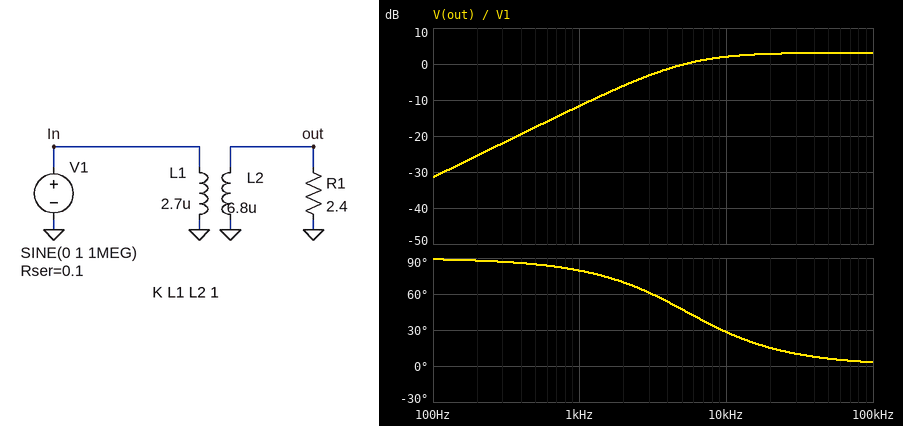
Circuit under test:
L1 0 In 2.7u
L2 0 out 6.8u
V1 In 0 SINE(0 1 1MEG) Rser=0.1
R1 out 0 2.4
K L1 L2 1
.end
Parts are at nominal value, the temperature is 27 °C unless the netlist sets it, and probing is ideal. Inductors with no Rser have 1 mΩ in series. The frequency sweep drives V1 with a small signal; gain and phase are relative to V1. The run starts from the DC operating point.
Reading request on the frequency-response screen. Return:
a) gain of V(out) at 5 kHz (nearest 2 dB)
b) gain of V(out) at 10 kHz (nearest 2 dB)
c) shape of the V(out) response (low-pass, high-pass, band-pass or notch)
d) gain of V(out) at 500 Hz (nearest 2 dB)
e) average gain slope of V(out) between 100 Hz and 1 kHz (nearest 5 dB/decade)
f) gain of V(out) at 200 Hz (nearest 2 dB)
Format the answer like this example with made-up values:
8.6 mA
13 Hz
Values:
0 dB
2 dB
high-pass
-18 dB
20 dB/decade
-26 dB
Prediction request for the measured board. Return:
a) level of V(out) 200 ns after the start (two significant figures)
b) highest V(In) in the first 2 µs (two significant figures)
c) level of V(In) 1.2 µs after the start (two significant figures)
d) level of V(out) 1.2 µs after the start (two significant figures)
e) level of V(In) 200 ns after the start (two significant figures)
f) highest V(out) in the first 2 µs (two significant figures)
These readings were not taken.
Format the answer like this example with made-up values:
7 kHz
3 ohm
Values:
1.4 V
900 mV
860 mV
1.4 V
860 mV
1.4 V
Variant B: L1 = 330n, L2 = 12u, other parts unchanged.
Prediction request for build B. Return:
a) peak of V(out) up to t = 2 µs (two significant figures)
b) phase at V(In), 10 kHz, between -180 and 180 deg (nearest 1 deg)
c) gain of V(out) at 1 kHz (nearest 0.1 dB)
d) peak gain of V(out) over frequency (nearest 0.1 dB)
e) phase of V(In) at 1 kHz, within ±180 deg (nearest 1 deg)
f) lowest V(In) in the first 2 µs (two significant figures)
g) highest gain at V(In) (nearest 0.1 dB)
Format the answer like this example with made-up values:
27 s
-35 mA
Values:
2.3 V
60 deg
-18.2 dB
7.5 dB
62 deg
-410 mV
-7.9 dB
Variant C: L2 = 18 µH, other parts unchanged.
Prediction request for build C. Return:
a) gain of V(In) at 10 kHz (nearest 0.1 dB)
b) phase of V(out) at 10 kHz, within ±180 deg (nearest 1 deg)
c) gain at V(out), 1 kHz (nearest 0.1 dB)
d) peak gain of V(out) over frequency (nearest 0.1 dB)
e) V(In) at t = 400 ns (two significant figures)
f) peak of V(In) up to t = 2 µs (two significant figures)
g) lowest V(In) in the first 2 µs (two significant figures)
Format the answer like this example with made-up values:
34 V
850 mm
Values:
-3.0 dB
25 deg
-7.5 dB
6.1 dB
450 mV
780 mV
-790 mV
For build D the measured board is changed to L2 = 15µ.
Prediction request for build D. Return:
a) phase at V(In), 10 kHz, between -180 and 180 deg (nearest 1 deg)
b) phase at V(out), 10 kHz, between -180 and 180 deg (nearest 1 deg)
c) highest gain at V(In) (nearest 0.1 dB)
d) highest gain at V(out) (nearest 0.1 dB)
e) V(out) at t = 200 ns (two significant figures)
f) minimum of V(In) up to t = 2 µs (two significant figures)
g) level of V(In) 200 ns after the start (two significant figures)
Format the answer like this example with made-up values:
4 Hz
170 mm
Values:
25 deg
26 deg
-1.8 dB
5.6 dB
1.8 V
-820 mV
770 mV
